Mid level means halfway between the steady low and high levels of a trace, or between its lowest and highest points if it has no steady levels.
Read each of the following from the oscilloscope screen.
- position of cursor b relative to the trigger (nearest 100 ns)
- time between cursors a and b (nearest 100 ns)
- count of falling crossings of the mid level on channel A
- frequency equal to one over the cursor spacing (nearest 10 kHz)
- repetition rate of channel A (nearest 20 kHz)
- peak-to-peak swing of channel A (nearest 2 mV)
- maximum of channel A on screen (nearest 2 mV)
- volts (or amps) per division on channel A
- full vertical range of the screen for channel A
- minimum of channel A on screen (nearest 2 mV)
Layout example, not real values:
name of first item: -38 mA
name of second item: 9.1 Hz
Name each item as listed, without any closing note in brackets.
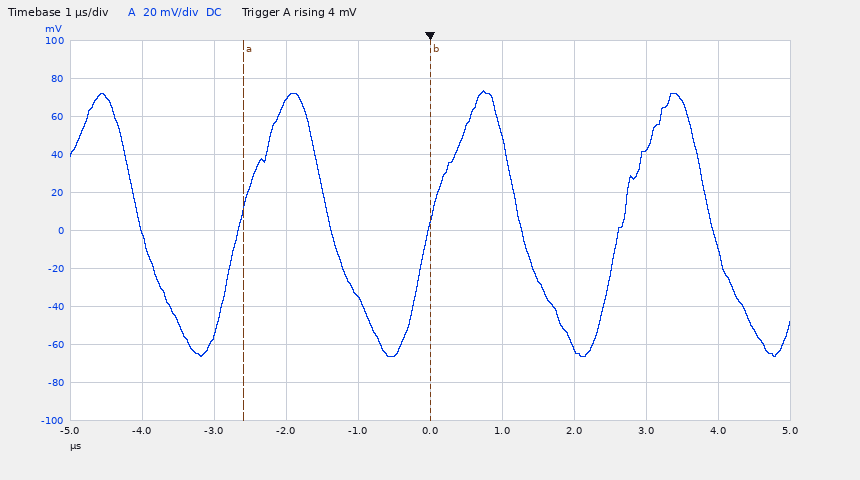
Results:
position of cursor b relative to the trigger: 0.0 µs
time between cursors a and b: 2.6 µs
count of falling crossings of the mid level on channel A: 4
frequency equal to one over the cursor spacing: 380 kHz
repetition rate of channel A: 380 kHz
peak-to-peak swing of channel A: 140 mV
maximum of channel A on screen: 74 mV
volts (or amps) per division on channel A: 20 mV
full vertical range of the screen for channel A: 200 mV
minimum of channel A on screen: -66 mV
